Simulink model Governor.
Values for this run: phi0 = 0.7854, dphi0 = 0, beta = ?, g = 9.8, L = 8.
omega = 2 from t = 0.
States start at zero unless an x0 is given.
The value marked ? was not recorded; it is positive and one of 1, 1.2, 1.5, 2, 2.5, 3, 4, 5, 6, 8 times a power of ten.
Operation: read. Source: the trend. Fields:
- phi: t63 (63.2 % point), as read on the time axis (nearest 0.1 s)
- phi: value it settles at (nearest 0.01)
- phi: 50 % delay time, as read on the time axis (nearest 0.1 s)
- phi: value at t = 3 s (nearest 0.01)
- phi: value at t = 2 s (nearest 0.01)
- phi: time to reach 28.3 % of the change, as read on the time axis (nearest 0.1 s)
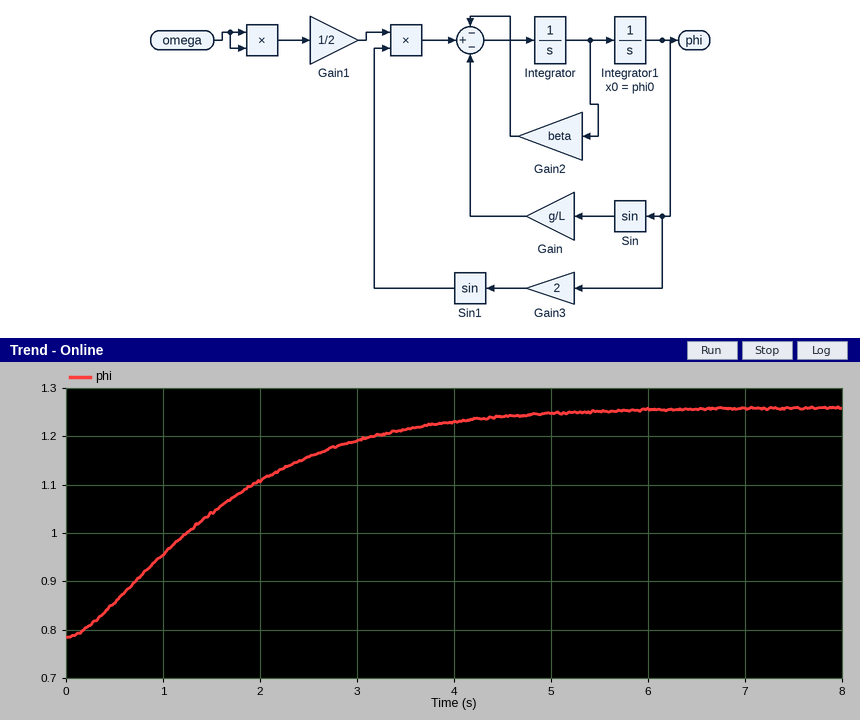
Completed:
1.8 s
1.26
1.4 s
1.19
1.11
0.8 s
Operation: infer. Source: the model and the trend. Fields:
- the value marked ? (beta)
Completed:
5
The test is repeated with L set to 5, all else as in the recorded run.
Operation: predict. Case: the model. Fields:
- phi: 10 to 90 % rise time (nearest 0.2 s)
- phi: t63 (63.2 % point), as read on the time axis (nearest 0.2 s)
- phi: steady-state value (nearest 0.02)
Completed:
3.6 s
2.0 s
1.06
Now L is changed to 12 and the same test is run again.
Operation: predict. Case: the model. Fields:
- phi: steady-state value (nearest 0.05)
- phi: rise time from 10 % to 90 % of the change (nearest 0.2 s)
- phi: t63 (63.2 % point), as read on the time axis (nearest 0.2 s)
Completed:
1.35
2.8 s
1.8 s
